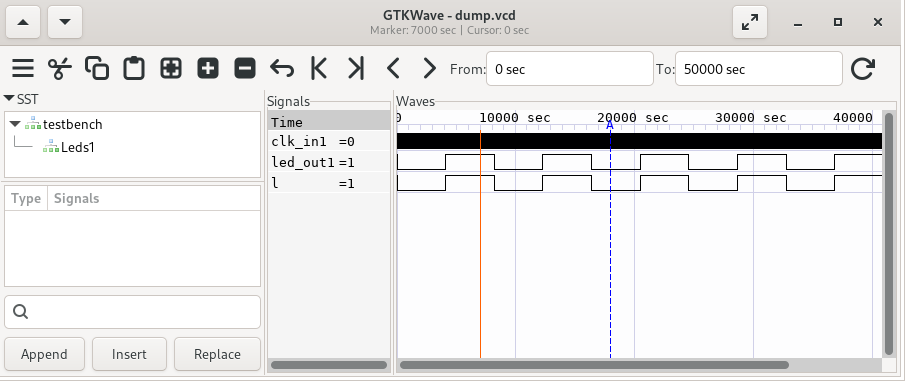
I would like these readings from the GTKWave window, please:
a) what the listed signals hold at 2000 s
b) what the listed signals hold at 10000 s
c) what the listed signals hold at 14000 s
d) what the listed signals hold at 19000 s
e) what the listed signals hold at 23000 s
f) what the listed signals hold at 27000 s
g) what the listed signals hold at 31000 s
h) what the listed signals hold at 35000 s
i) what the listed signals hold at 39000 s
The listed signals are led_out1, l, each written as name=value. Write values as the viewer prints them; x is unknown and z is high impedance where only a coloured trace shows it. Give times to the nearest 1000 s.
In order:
led_out1=0, l=0
led_out1=0, l=0
led_out1=1, l=1
led_out1=0, l=0
led_out1=1, l=1
led_out1=0, l=0
led_out1=1, l=1
led_out1=0, l=0
led_out1=1, l=1
